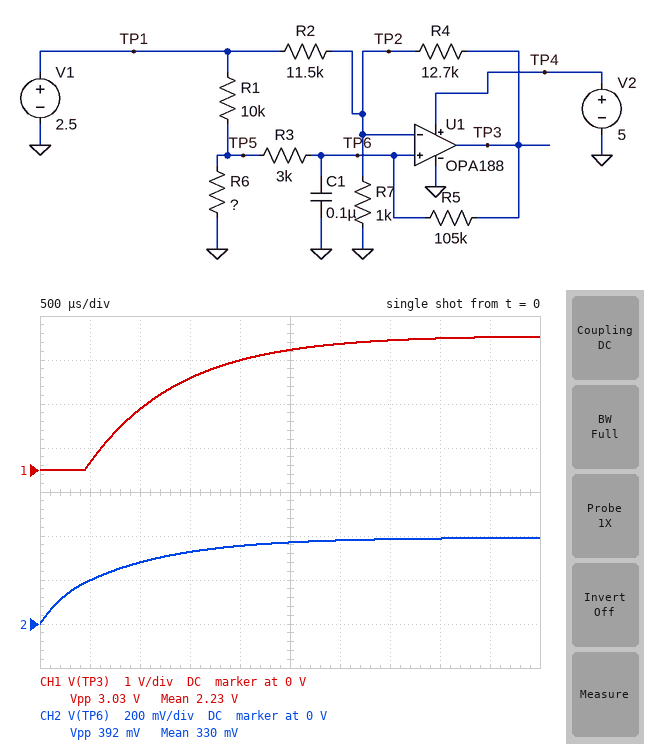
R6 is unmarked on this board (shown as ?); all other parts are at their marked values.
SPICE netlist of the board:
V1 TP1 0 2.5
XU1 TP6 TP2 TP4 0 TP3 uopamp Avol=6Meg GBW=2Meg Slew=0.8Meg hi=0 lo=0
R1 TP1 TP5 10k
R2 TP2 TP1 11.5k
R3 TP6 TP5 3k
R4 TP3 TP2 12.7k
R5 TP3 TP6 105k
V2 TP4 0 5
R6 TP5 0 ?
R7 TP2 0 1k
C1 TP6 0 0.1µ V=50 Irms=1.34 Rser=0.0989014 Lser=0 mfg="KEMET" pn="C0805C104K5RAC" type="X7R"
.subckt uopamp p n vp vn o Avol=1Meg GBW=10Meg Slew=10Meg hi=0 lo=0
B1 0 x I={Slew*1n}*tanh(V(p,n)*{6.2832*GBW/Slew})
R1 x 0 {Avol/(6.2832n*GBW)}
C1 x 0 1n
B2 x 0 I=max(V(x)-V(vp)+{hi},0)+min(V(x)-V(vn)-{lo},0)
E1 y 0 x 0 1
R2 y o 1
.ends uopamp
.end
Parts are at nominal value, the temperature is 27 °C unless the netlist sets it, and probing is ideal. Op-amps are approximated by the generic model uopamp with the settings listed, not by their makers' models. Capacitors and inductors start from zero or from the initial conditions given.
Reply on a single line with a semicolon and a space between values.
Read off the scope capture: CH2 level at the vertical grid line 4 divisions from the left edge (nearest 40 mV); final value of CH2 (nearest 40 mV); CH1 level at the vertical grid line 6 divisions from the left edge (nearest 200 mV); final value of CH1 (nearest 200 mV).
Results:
360 mV; 400 mV; 2.8 V; 3.0 V
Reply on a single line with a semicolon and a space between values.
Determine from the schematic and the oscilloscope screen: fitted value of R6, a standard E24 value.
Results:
1.3 kΩ
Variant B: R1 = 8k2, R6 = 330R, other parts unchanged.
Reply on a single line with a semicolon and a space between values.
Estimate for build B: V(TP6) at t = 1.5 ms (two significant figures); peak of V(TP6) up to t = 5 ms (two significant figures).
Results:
93 mV; 94 mV
